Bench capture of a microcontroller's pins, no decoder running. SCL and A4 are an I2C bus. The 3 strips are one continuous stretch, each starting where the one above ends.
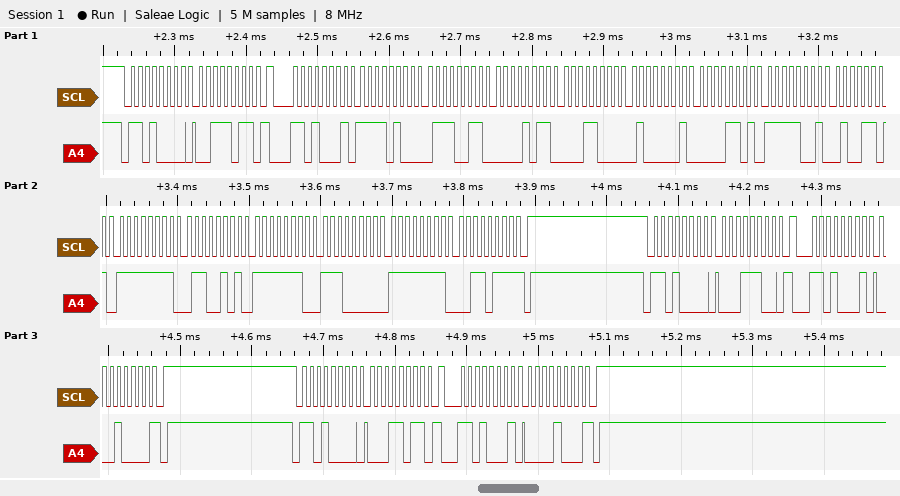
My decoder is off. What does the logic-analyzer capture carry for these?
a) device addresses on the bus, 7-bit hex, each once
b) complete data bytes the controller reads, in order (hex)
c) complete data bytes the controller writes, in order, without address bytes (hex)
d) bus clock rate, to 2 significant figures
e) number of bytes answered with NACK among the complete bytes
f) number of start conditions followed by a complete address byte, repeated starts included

0x68
F4 73 0B 18 41 0D F9 4D FF 65 FE E0 FF 37 10 08
3B 1C 1B
100 kHz
3
6
